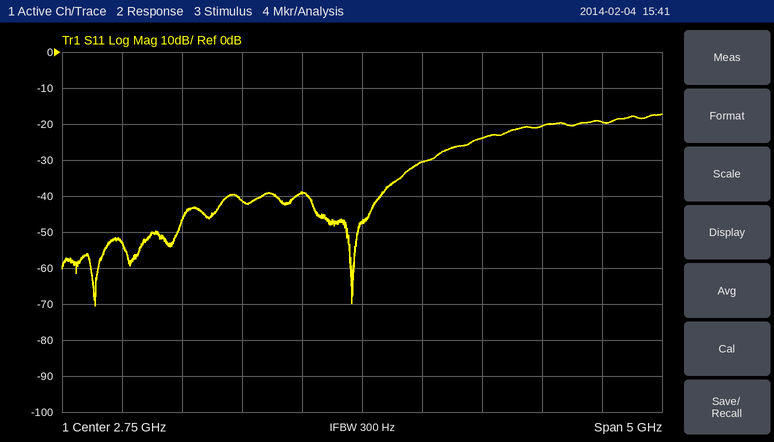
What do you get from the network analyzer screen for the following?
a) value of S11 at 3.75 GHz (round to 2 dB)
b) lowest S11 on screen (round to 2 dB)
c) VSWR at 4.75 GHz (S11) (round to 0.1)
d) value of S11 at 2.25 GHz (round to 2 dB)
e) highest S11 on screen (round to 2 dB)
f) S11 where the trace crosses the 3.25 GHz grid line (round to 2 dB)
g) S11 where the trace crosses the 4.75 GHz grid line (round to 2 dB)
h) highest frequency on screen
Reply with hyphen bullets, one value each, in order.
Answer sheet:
- -24 dB
- -70 dB
- 1.2
- -40 dB
- -18 dB
- -30 dB
- -20 dB
- 5.25 GHz
